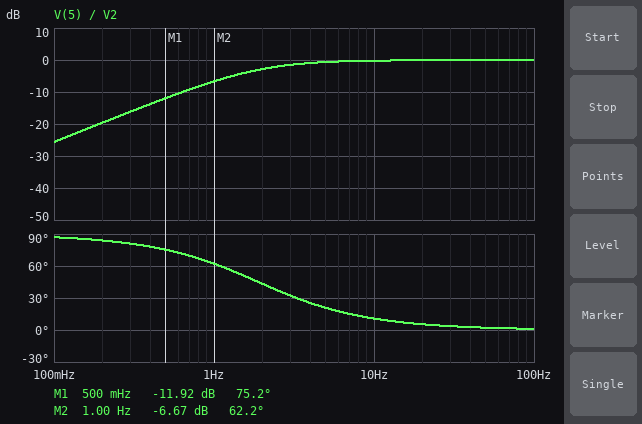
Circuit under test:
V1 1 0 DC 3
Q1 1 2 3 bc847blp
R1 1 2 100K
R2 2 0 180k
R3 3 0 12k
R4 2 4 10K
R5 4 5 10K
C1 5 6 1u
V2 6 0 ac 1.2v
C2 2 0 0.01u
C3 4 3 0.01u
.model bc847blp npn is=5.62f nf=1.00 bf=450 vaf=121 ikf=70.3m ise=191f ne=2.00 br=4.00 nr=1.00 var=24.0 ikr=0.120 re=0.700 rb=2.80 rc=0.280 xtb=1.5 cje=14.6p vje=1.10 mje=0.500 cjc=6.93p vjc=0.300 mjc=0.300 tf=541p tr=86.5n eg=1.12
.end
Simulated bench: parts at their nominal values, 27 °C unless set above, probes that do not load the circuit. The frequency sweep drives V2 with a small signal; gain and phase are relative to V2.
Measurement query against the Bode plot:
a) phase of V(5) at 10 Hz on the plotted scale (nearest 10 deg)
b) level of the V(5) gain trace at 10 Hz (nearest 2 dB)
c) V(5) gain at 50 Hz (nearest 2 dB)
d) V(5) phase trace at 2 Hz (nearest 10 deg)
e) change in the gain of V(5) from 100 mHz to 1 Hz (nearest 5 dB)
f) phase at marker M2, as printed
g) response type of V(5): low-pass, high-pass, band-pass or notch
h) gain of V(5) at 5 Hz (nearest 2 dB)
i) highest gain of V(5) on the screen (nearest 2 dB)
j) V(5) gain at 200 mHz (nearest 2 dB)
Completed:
10 deg
0 dB
0 dB
40 deg
20 dB
62.2 deg
high-pass
0 dB
0 dB
-20 dB
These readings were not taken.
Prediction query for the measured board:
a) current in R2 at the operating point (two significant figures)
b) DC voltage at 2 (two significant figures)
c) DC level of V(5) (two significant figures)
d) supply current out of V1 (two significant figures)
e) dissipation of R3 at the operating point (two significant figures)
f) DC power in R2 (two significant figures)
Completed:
11 µA
1.9 V
1.9 V
120 µA
140 µW
20 µW
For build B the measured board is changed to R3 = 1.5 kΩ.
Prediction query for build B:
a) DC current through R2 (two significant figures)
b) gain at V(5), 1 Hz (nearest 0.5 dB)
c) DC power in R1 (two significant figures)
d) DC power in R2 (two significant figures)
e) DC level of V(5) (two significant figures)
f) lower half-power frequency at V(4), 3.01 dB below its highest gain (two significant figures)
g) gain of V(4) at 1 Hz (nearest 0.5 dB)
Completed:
10 µA
-7.0 dB
14 µW
18 µW
1.8 V
2.0 Hz
-8.5 dB
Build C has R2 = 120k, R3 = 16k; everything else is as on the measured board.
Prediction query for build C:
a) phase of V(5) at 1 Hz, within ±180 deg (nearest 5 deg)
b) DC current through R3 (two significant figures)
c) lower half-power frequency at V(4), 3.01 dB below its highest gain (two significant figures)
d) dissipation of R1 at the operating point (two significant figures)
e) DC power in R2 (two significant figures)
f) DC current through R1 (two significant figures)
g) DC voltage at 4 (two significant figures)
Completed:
65 deg
64 µA
2.1 Hz
19 µW
22 µW
14 µA
1.6 V
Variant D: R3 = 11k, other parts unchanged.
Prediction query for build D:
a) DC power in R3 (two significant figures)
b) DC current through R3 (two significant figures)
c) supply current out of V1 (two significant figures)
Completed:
150 µW
120 µA
130 µA
